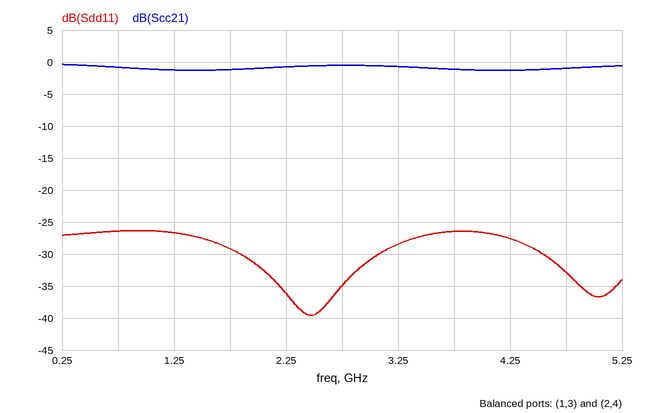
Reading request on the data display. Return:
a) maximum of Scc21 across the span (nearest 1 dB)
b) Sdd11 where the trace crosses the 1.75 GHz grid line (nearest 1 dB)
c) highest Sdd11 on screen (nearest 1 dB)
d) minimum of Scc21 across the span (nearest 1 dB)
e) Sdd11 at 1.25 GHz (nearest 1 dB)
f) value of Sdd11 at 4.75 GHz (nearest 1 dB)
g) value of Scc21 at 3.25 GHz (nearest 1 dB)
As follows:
0 dB
-29 dB
-26 dB
-1 dB
-27 dB
-33 dB
-1 dB
